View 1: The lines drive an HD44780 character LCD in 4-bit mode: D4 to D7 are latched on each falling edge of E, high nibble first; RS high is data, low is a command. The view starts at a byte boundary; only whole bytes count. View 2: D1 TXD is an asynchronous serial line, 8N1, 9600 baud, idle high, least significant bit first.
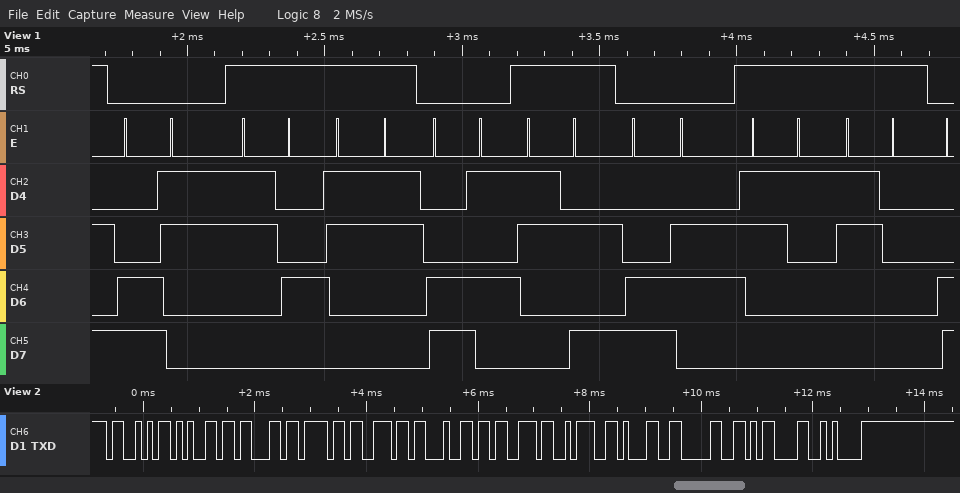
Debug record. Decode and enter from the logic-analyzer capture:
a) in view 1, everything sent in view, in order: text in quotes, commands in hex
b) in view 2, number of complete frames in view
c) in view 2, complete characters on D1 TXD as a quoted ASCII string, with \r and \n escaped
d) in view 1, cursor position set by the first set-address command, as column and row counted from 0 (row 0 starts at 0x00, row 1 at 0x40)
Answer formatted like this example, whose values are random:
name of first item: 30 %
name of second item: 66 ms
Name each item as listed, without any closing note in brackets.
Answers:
in view 1, everything sent in view, in order: text in quotes, commands in hex: 0xC3 "43" 0xC5 ":" 0xC6 "10"
in view 2, number of complete frames in view: 12
in view 2, complete characters on D1 TXD as a quoted ASCII string, with \r and \n escaped: "Seconds:10\r\n"
in view 1, cursor position set by the first set-address command, as column and row counted from 0: column 3, row 1
